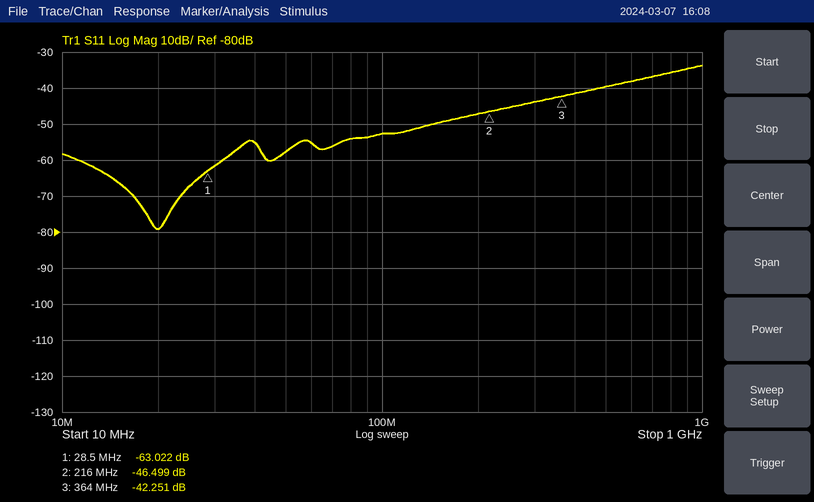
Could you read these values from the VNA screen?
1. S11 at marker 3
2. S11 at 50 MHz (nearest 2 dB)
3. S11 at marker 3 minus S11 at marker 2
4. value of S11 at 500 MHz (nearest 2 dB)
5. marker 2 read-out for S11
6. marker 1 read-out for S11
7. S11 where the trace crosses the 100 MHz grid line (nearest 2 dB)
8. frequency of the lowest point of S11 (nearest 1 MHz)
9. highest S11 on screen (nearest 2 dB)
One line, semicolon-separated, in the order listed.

-42.251 dB; -58 dB; 4.248 dB; -40 dB; -46.499 dB; -63.022 dB; -52 dB; 20 MHz; -34 dB
